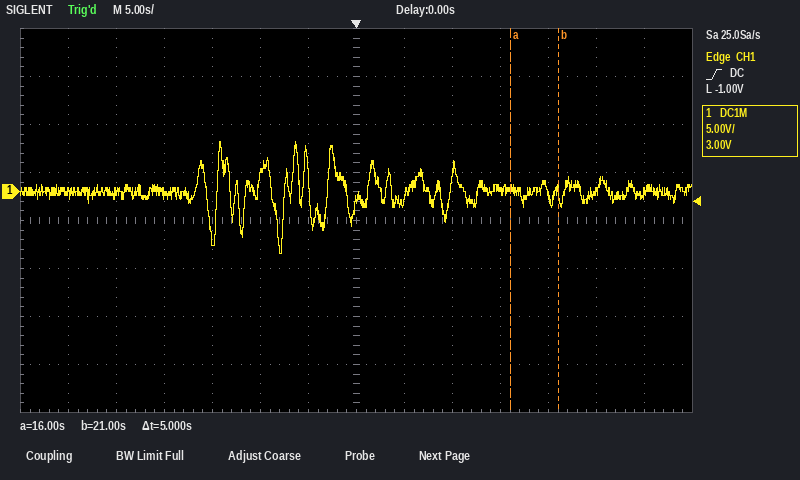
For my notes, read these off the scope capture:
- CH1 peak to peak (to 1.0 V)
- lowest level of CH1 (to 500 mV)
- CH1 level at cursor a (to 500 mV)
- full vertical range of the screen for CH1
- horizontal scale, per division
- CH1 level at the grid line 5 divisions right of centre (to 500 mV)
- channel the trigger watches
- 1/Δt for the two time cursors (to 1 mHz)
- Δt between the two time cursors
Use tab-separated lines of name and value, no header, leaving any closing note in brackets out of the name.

CH1 peak to peak	12.0 V
lowest level of CH1	-6.5 V
CH1 level at cursor a	500 mV
full vertical range of the screen for CH1	40 V
horizontal scale, per division	5 s
CH1 level at the grid line 5 divisions right of centre	0.0 V
channel the trigger watches	CH1
1/Δt for the two time cursors	200 mHz
Δt between the two time cursors	5 s
